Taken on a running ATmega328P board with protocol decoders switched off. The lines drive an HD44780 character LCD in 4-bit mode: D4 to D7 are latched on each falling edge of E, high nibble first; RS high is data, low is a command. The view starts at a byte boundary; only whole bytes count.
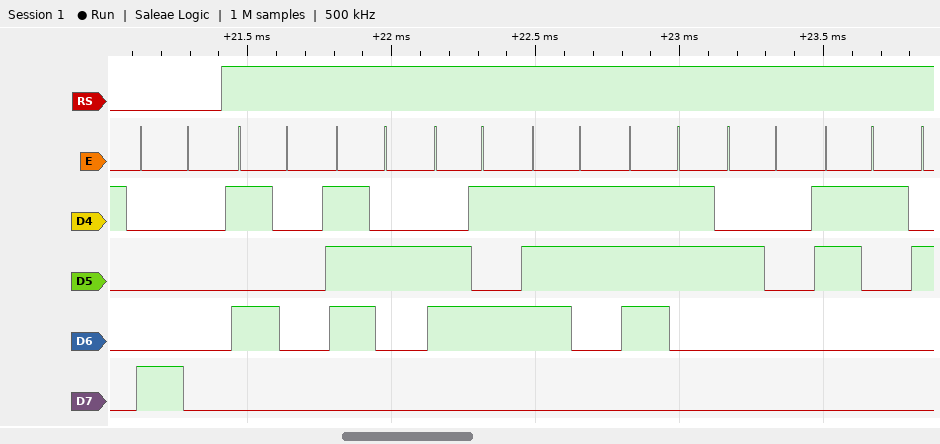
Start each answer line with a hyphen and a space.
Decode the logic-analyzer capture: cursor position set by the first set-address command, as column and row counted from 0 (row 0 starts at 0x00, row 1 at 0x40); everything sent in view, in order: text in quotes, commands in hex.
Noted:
- column 0, row 0
- 0x80 "Press 1"
